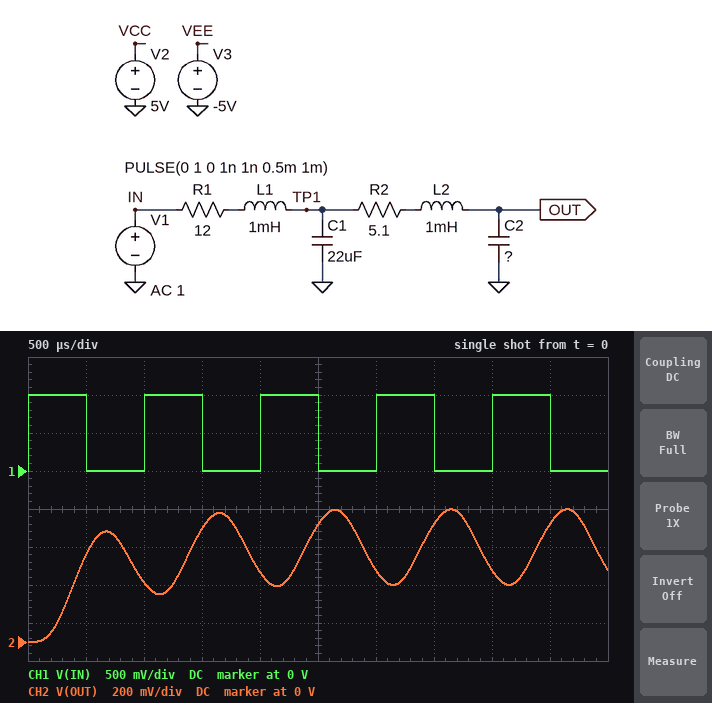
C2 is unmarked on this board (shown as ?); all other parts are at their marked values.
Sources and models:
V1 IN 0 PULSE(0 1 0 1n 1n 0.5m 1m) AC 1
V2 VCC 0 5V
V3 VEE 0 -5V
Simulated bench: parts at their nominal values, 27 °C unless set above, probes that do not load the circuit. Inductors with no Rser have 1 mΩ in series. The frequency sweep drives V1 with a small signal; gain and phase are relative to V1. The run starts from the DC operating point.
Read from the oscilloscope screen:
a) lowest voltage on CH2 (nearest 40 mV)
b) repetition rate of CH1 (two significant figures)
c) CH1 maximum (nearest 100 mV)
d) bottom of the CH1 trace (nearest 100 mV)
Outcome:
0 V
1.0 kHz
1.0 V
0 V
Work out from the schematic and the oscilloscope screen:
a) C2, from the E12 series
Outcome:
27 µF
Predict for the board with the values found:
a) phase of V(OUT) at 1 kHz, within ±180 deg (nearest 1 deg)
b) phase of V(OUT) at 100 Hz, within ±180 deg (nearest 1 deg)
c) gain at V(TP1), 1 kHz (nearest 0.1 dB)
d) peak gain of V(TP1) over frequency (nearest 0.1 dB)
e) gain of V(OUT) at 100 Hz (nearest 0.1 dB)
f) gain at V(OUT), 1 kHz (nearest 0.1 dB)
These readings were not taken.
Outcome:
-141 deg
-25 deg
-11.4 dB
0 dB
-0.5 dB
-10.2 dB
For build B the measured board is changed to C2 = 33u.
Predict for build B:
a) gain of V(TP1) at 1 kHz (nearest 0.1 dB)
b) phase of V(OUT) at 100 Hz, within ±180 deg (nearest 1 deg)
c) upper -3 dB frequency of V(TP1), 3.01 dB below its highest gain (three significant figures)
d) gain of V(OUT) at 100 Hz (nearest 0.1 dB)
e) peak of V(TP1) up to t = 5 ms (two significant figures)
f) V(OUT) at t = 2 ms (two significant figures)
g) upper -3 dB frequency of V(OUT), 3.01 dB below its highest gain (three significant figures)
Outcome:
-10.7 dB
-29 deg
228 Hz
-0.7 dB
670 mV
390 mV
246 Hz
